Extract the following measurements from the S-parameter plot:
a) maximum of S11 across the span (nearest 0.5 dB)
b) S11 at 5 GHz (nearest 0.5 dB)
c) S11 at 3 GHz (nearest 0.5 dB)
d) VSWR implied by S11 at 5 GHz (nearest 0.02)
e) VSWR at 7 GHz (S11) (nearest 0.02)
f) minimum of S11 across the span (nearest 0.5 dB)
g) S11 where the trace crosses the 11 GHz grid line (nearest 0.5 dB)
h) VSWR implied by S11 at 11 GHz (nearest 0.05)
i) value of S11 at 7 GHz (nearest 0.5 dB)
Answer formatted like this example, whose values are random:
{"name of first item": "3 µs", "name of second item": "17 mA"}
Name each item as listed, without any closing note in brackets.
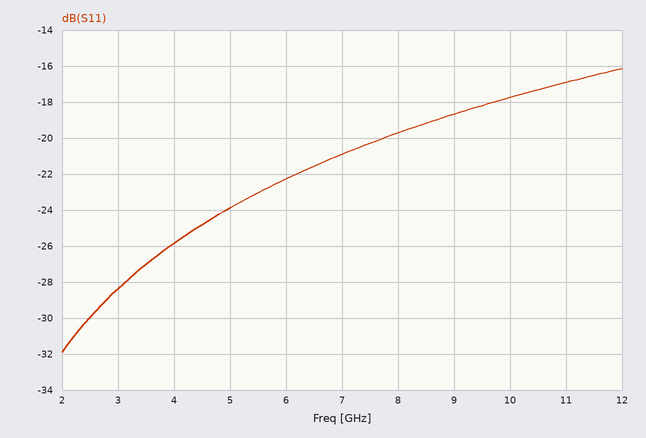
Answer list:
{"maximum of S11 across the span": "-16.0 dB", "S11 at 5 GHz": "-24.0 dB", "S11 at 3 GHz": "-28.5 dB", "VSWR implied by S11 at 5 GHz": "1.14", "VSWR at 7 GHz (S11)": "1.20", "minimum of S11 across the span": "-32.0 dB", "S11 where the trace crosses the 11 GHz grid line": "-17.0 dB", "VSWR implied by S11 at 11 GHz": "1.35", "value of S11 at 7 GHz": "-21.0 dB"}
